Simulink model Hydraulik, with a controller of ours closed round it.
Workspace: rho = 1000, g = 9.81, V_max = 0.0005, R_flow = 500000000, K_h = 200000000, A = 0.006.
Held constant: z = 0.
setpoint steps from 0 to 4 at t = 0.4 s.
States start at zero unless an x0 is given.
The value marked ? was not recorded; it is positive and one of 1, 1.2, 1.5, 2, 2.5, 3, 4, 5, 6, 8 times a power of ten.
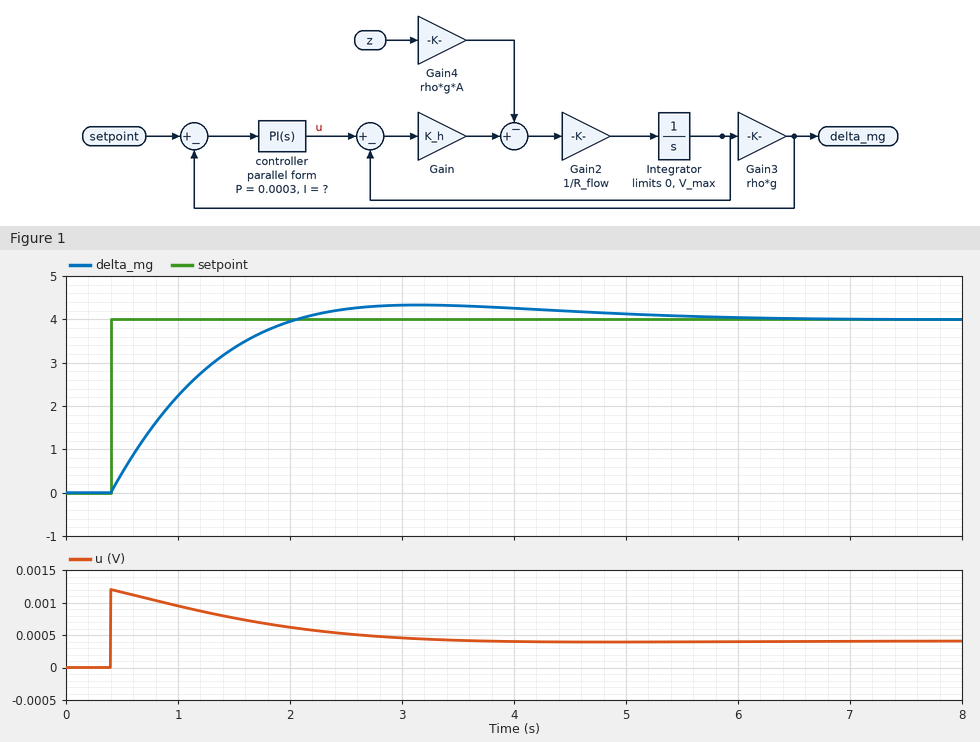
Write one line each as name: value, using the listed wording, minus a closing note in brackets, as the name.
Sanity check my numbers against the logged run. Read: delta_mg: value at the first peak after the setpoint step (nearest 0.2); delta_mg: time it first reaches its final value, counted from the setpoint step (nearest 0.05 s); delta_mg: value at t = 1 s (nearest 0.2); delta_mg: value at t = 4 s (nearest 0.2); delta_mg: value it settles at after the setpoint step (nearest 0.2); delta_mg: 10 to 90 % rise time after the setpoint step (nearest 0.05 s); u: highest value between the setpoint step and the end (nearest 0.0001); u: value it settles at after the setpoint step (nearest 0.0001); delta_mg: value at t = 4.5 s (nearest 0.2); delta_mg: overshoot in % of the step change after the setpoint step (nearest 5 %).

delta_mg: value at the first peak after the setpoint step: 4.4
delta_mg: time it first reaches its final value, counted from the setpoint step: 1.65 s
delta_mg: value at t = 1 s: 2.2
delta_mg: value at t = 4 s: 4.2
delta_mg: value it settles at after the setpoint step: 4.0
delta_mg: 10 to 90 % rise time after the setpoint step: 1.20 s
u: highest value between the setpoint step and the end: 0.0012
u: value it settles at after the setpoint step: 0.0004
delta_mg: value at t = 4.5 s: 4.2
delta_mg: overshoot in % of the step change after the setpoint step: 10 %
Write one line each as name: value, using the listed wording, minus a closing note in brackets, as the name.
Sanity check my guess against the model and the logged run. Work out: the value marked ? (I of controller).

the value marked ?: 0.00025
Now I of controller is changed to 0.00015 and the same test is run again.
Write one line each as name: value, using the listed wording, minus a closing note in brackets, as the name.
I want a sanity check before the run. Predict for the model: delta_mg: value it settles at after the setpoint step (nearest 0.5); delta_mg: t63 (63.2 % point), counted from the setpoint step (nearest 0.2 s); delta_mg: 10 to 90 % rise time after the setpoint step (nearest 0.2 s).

delta_mg: value it settles at after the setpoint step: 4.0
delta_mg: t63 (63.2 % point), counted from the setpoint step: 0.8 s
delta_mg: 10 to 90 % rise time after the setpoint step: 1.6 s
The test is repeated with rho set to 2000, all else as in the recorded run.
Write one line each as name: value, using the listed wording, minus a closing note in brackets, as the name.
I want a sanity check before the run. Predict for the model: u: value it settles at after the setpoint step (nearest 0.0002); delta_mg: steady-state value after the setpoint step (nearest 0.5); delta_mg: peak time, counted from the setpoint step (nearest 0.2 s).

u: value it settles at after the setpoint step: 0.0002
delta_mg: steady-state value after the setpoint step: 4.0
delta_mg: peak time, counted from the setpoint step: 1.8 s
